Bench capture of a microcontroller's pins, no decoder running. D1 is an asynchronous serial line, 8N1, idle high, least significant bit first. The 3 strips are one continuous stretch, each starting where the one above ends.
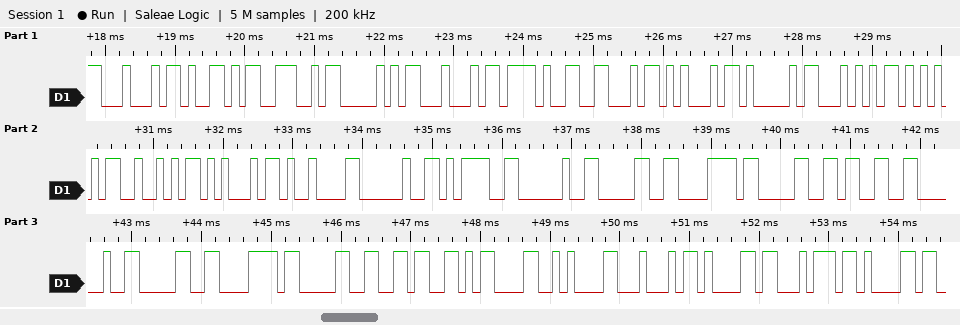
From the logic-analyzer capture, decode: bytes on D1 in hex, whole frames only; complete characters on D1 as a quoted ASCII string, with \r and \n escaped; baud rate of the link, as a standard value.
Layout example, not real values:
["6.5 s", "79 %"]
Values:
["44 59 4E 50 44 2F 46 45 41 54 55 52 45 09 20 3D 20 30 78 30 33 20 30 78 30 36 0D 0A 44 61 74 61", "\"DYNPD/FEATURE\\t = 0x03 0x06\\r\\nData\"", "9600 baud"]
